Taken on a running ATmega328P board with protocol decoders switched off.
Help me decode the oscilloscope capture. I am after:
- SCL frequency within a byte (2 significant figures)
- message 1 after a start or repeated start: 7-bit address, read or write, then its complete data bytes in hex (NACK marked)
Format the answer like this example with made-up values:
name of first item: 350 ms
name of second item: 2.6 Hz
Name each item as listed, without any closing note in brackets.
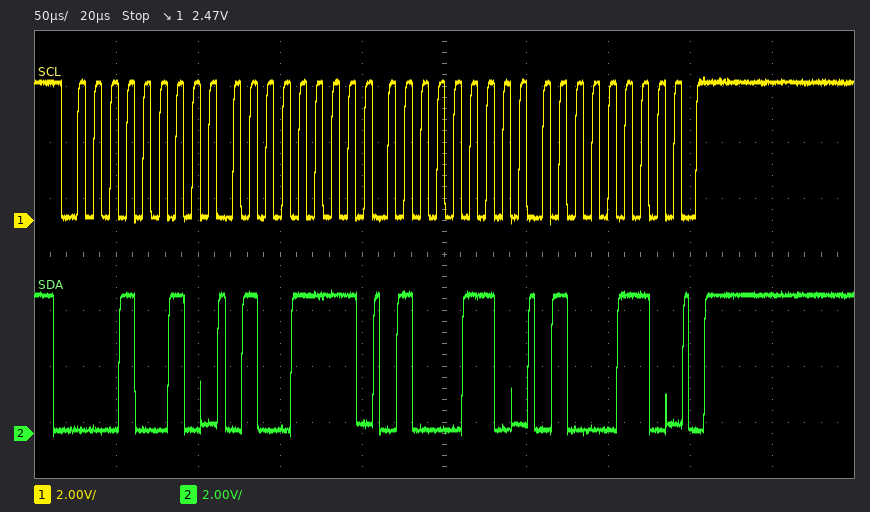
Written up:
SCL frequency within a byte: 100 kHz
message 1 after a start or repeated start: 7-bit address, read or write, then its complete data bytes in hex: 0x09 write: 4F 46 46
